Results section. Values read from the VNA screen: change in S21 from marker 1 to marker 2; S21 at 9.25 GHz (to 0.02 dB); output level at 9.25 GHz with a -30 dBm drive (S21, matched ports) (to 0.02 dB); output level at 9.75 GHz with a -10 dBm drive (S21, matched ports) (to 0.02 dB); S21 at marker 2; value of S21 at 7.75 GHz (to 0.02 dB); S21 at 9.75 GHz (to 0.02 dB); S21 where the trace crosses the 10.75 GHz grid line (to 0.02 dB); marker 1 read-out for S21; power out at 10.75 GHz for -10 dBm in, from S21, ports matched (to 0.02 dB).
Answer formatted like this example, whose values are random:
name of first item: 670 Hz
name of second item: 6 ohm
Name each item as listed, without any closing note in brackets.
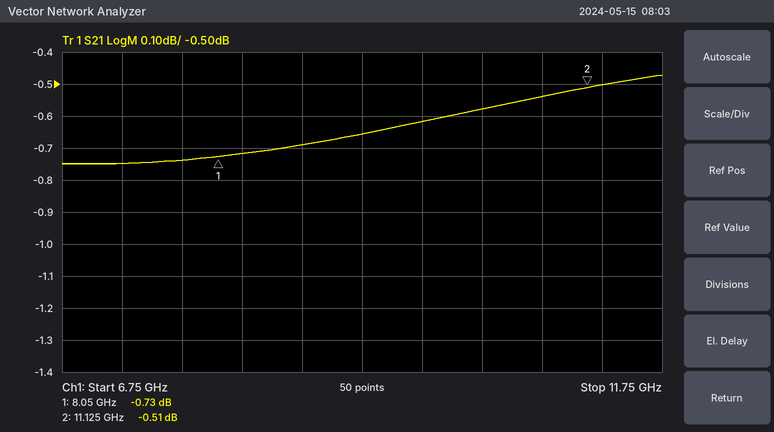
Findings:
change in S21 from marker 1 to marker 2: 0.22 dB
S21 at 9.25 GHz: -0.66 dB
output level at 9.25 GHz with a -30 dBm drive (S21, matched ports): -30.66 dBm
output level at 9.75 GHz with a -10 dBm drive (S21, matched ports): -10.62 dBm
S21 at marker 2: -0.51 dB
value of S21 at 7.75 GHz: -0.74 dB
S21 at 9.75 GHz: -0.62 dB
S21 where the trace crosses the 10.75 GHz grid line: -0.54 dB
marker 1 read-out for S21: -0.73 dB
power out at 10.75 GHz for -10 dBm in, from S21, ports matched: -10.54 dBm
